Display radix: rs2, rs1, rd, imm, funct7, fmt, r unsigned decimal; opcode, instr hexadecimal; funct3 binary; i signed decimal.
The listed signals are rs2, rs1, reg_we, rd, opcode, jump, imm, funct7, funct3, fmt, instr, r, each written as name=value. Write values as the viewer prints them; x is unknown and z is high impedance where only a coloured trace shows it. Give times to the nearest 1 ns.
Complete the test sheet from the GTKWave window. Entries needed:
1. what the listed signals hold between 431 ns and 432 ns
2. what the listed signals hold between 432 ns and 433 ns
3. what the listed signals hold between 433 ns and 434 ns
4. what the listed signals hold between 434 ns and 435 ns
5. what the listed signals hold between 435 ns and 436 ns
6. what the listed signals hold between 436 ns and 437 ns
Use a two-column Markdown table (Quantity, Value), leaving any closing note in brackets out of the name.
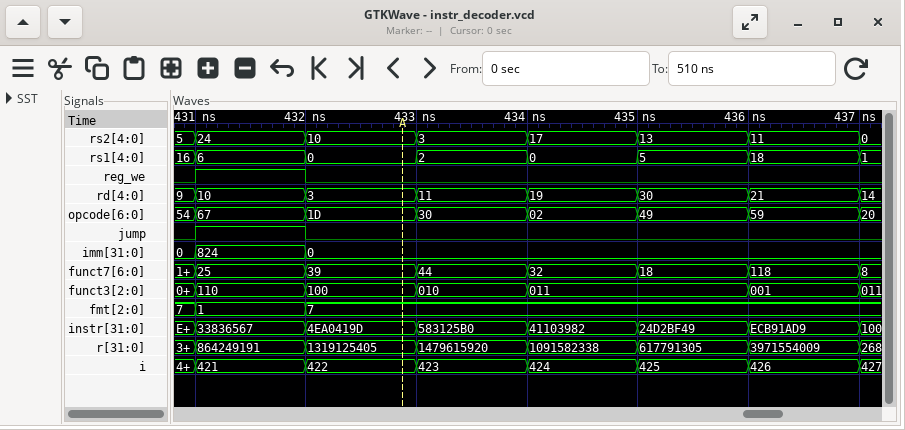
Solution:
| Quantity | Value |
|---|---|
| what the listed signals hold between 431 ns and 432 ns | rs2=24, rs1=6, reg_we=1, rd=10, opcode=67, jump=1, imm=824, funct7=25, funct3=110, fmt=1, instr=33836567, r=864249191 |
| what the listed signals hold between 432 ns and 433 ns | rs2=10, rs1=0, reg_we=0, rd=3, opcode=1D, jump=0, imm=0, funct7=39, funct3=100, fmt=7, instr=4EA0419D, r=1319125405 |
| what the listed signals hold between 433 ns and 434 ns | rs2=3, rs1=2, reg_we=0, rd=11, opcode=30, jump=0, imm=0, funct7=44, funct3=010, fmt=7, instr=583125B0, r=1479615920 |
| what the listed signals hold between 434 ns and 435 ns | rs2=17, rs1=0, reg_we=0, rd=19, opcode=02, jump=0, imm=0, funct7=32, funct3=011, fmt=7, instr=41103982, r=1091582338 |
| what the listed signals hold between 435 ns and 436 ns | rs2=13, rs1=5, reg_we=0, rd=30, opcode=49, jump=0, imm=0, funct7=18, funct3=011, fmt=7, instr=24D2BF49, r=617791305 |
| what the listed signals hold between 436 ns and 437 ns | rs2=11, rs1=18, reg_we=0, rd=21, opcode=59, jump=0, imm=0, funct7=118, funct3=001, fmt=7, instr=ECB91AD9, r=3971554009 |
